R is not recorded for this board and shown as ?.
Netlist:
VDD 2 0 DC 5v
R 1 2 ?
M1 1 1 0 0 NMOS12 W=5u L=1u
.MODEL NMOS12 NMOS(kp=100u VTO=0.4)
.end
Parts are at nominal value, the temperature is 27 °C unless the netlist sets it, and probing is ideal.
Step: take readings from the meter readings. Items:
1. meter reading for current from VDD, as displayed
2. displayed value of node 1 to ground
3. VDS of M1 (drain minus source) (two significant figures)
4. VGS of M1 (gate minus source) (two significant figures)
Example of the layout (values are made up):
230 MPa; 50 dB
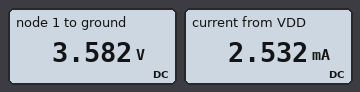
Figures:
2.532 mA; 3.582 V; 3.6 V; 3.6 V
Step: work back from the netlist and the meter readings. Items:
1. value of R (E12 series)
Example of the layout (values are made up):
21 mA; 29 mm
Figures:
560 Ω
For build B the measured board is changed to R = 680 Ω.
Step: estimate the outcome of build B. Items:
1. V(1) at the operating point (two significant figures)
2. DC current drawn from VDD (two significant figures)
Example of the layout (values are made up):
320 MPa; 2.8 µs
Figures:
3.4 V; 2.3 mA
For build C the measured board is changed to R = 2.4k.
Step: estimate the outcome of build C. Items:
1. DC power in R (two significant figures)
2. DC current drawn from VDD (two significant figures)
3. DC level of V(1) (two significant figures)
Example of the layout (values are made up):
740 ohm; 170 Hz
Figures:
2.7 mW; 1.1 mA; 2.5 V
